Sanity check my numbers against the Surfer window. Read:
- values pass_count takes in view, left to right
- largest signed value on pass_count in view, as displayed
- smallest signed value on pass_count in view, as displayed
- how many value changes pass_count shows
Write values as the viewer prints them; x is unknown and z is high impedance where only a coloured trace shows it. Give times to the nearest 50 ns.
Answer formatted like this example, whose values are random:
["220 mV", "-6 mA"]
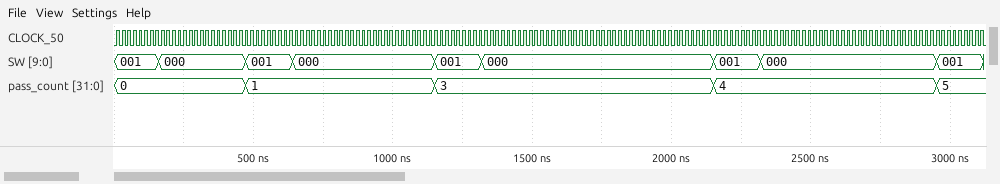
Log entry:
["0, 1, 3, 4, 5", "5", "0", "4"]
